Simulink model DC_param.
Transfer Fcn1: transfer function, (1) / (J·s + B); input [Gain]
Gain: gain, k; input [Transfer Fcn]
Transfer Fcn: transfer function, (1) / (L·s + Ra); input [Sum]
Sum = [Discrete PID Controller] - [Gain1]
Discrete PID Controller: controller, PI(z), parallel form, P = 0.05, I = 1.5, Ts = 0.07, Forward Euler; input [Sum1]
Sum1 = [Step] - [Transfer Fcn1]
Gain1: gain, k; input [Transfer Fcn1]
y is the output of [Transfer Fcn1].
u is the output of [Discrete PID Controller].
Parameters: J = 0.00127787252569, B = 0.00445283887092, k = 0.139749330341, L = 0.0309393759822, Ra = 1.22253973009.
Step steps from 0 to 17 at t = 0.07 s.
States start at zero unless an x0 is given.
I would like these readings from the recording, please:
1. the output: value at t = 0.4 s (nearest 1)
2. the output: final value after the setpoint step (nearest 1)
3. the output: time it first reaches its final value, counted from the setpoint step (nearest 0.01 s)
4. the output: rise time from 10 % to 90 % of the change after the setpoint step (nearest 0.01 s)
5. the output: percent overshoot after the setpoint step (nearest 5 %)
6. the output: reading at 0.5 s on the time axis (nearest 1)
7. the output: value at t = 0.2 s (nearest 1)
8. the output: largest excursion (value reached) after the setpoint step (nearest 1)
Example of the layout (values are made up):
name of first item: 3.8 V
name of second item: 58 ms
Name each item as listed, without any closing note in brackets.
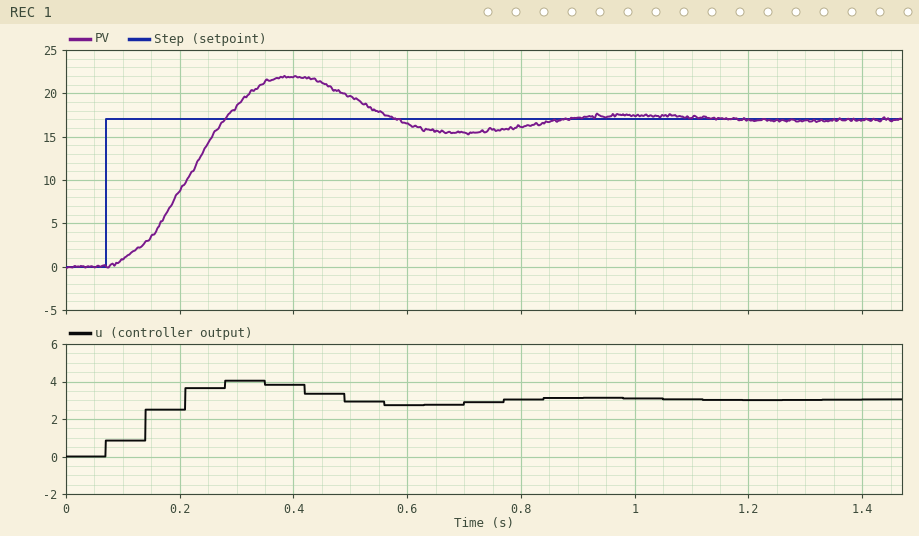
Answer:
the output: value at t = 0.4 s: 22
the output: final value after the setpoint step: 17
the output: time it first reaches its final value, counted from the setpoint step: 0.21 s
the output: rise time from 10 % to 90 % of the change after the setpoint step: 0.14 s
the output: percent overshoot after the setpoint step: 30 %
the output: reading at 0.5 s on the time axis: 20
the output: value at t = 0.2 s: 9
the output: largest excursion (value reached) after the setpoint step: 22
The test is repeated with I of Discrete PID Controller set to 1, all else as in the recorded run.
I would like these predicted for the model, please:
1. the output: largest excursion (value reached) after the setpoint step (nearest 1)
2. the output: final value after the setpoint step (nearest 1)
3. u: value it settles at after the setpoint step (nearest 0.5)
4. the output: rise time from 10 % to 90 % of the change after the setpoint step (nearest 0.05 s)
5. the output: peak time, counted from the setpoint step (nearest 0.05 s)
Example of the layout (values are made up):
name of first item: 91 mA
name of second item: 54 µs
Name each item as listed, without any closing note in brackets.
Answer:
the output: largest excursion (value reached) after the setpoint step: 18
the output: final value after the setpoint step: 17
u: value it settles at after the setpoint step: 3.0
the output: rise time from 10 % to 90 % of the change after the setpoint step: 0.20 s
the output: peak time, counted from the setpoint step: 0.45 s
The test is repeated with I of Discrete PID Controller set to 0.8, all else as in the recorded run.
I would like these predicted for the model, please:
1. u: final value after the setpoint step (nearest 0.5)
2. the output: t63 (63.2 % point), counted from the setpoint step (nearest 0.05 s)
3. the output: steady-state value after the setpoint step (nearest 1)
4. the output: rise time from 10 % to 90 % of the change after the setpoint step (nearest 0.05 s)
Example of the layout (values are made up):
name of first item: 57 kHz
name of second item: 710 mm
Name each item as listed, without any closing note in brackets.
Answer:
u: final value after the setpoint step: 3.0
the output: t63 (63.2 % point), counted from the setpoint step: 0.20 s
the output: steady-state value after the setpoint step: 17
the output: rise time from 10 % to 90 % of the change after the setpoint step: 0.30 s
